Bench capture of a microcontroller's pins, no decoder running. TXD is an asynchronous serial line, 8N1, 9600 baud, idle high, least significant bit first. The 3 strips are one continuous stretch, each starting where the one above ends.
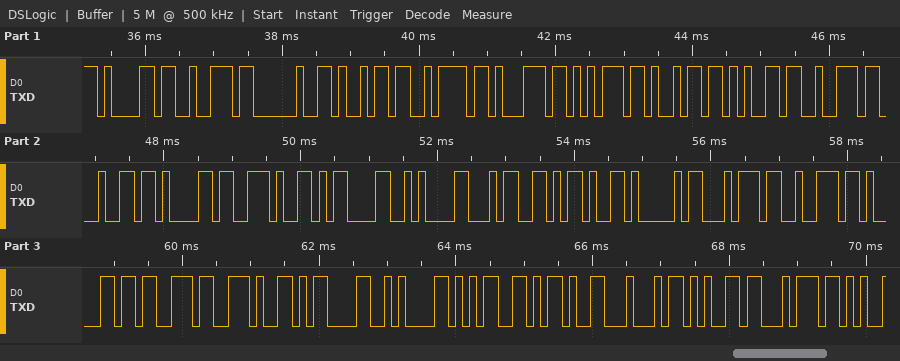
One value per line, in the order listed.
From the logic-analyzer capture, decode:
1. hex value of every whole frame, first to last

61 72 20 69 7A 71 75 69 65 72 64 61 2E 0D 0A 34 2D 41 74 72 61 73 2E 0D 0A 35 2D 44 65 74
